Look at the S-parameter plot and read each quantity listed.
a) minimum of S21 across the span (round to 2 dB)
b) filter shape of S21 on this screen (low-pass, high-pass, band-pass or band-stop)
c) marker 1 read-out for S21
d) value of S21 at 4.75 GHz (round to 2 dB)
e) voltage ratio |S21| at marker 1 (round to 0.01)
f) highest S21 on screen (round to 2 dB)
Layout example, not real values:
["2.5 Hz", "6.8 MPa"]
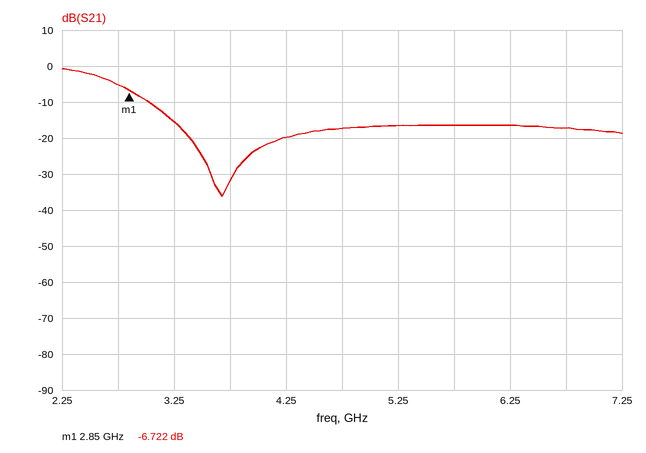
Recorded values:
["-36 dB", "low-pass", "-6.722 dB", "-18 dB", "0.46", "0 dB"]
